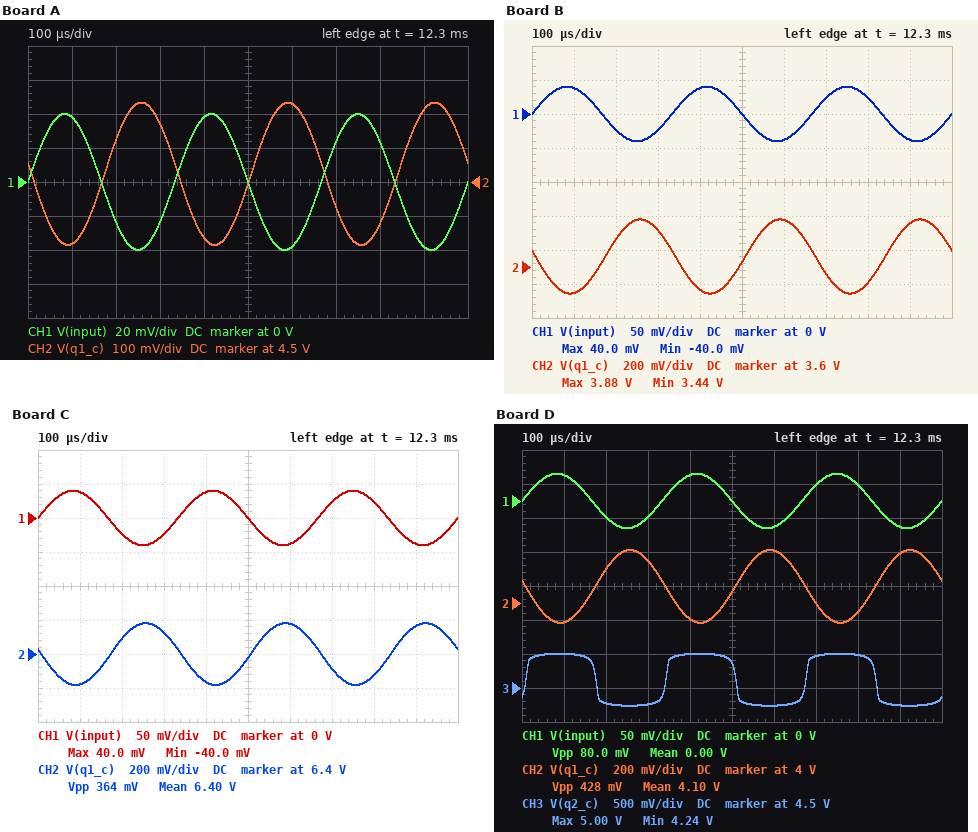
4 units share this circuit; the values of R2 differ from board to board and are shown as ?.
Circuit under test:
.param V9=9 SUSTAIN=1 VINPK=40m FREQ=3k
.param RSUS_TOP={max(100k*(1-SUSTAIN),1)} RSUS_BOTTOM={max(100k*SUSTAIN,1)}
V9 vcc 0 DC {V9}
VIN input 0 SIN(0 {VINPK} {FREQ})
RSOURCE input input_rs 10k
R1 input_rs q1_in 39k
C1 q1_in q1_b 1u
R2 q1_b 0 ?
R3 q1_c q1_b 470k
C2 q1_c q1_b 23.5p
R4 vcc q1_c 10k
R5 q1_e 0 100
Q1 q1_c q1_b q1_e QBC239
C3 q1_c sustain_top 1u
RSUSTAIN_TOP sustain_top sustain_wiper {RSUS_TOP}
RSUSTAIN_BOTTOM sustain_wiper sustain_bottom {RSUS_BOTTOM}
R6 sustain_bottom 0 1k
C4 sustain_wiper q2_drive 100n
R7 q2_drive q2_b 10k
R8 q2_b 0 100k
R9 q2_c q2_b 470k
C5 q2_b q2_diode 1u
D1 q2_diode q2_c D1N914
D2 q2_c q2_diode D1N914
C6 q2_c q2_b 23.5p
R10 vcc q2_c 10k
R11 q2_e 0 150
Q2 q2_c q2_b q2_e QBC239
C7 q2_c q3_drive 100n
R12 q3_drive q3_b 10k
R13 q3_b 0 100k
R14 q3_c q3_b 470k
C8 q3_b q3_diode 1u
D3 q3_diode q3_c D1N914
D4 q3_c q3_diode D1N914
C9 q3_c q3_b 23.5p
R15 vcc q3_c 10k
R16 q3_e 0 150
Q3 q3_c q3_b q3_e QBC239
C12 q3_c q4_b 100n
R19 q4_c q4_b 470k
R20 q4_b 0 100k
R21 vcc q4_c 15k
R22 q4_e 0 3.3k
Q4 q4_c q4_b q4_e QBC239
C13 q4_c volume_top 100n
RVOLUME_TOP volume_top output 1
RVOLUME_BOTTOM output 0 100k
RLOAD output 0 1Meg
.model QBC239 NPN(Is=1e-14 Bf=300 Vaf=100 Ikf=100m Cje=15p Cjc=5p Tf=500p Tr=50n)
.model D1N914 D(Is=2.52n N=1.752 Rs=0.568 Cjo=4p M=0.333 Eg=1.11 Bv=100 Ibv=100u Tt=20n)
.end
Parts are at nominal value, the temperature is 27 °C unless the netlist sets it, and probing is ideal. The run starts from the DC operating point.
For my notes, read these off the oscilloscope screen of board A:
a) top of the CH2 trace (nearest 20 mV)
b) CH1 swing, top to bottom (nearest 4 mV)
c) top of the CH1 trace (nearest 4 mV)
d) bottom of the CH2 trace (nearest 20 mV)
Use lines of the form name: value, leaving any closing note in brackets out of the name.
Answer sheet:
top of the CH2 trace: 4.74 V
CH1 swing, top to bottom: 80 mV
top of the CH1 trace: 40 mV
bottom of the CH2 trace: 4.32 V
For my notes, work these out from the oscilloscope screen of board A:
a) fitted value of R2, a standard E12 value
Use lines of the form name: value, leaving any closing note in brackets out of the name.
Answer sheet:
fitted value of R2, a standard E12 value: 100 kΩ
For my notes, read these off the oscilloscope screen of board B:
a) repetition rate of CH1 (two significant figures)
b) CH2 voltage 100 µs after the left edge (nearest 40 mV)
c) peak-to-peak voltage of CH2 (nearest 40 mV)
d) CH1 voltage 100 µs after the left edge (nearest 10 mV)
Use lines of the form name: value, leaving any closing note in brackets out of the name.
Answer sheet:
repetition rate of CH1: 3.0 kHz
CH2 voltage 100 µs after the left edge: 3.44 V
peak-to-peak voltage of CH2: 440 mV
CH1 voltage 100 µs after the left edge: 40 mV
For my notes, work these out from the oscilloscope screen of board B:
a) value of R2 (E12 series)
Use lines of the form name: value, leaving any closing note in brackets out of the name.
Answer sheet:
value of R2: 150 kΩ
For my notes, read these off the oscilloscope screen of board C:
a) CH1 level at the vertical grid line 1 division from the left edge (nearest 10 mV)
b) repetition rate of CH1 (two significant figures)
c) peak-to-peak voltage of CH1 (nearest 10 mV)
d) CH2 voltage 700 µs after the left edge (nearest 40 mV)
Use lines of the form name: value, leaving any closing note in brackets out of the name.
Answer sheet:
CH1 level at the vertical grid line 1 division from the left edge: 40 mV
repetition rate of CH1: 3.0 kHz
peak-to-peak voltage of CH1: 80 mV
CH2 voltage 700 µs after the left edge: 6.32 V
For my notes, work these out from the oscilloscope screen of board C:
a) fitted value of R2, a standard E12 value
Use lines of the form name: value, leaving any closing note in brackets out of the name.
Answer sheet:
fitted value of R2, a standard E12 value: 56 kΩ
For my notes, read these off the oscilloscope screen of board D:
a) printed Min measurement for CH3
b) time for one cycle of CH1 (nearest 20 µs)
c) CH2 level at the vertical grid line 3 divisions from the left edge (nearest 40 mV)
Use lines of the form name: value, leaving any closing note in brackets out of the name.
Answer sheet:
printed Min measurement for CH3: 4.24 V
time for one cycle of CH1: 340 µs
CH2 level at the vertical grid line 3 divisions from the left edge: 4.24 V
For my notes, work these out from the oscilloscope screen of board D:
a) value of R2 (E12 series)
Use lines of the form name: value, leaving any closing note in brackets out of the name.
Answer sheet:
value of R2: 120 kΩ
